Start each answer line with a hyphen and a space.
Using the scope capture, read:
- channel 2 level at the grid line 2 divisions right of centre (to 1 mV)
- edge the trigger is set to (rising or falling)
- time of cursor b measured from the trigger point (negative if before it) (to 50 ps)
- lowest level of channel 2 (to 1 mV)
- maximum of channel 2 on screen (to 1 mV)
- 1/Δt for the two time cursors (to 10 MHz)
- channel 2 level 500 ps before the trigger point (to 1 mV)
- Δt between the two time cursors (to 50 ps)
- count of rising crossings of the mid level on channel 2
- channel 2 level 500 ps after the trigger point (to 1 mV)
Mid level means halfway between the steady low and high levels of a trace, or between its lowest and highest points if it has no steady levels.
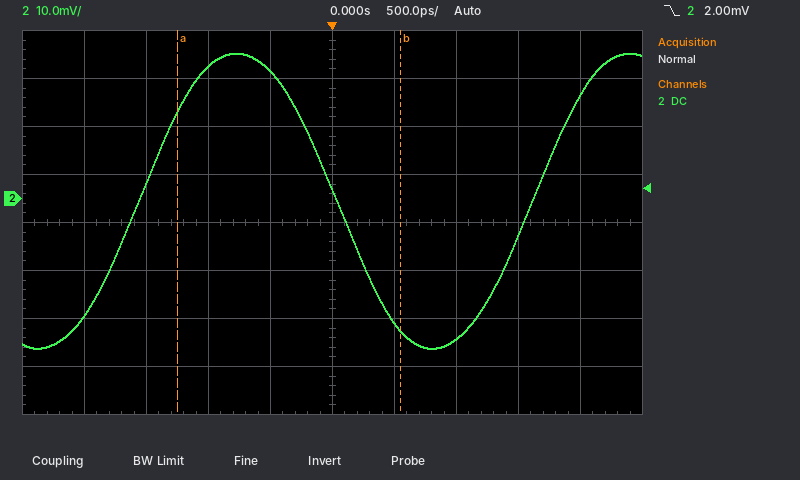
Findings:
- -29 mV
- falling
- +550 ps
- -31 mV
- 30 mV
- 560 MHz
- 27 mV
- 1.80 ns
- 2
- -26 mV
